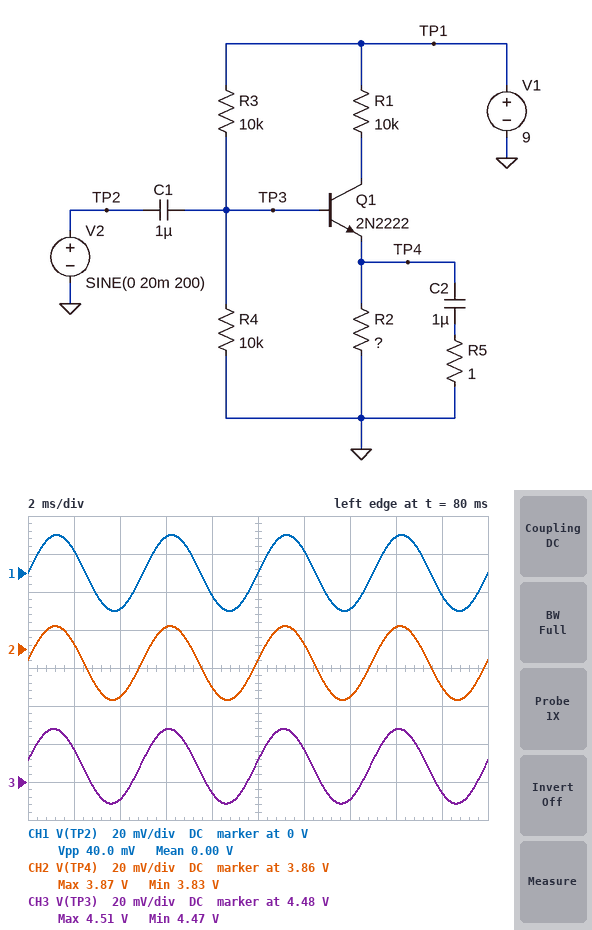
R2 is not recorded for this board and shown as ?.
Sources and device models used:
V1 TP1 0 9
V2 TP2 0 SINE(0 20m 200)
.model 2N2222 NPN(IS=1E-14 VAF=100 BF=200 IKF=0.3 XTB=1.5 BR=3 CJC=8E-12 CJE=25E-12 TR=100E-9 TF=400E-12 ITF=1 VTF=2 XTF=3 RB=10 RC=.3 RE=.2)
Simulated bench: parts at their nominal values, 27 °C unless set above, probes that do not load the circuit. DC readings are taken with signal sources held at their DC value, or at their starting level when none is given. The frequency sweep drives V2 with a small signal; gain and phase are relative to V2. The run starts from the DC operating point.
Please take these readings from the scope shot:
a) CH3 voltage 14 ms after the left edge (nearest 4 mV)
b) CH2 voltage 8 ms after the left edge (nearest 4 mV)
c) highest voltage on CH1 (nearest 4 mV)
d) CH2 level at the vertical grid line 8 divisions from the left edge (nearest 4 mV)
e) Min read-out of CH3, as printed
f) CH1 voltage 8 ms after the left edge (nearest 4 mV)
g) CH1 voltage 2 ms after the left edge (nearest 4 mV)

4.472 V
3.840 V
20 mV
3.872 V
4.47 V
-12 mV
12 mV
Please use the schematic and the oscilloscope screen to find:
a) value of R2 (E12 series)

8.2 kΩ
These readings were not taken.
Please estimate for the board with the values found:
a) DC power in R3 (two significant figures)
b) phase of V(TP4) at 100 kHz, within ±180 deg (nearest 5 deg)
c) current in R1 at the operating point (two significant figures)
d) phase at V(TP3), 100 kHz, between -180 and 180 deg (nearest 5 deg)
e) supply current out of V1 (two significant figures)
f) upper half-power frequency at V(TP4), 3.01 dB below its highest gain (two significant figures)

2.0 mW
-55 deg
470 µA
0 deg
920 µA
2.8 kHz
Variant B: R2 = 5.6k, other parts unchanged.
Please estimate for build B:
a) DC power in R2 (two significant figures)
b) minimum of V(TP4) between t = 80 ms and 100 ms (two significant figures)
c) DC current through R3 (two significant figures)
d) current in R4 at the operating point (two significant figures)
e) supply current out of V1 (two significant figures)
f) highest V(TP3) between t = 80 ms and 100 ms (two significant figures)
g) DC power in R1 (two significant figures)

2.2 mW
3.5 V
490 µA
410 µA
1.0 mA
4.1 V
3.0 mW
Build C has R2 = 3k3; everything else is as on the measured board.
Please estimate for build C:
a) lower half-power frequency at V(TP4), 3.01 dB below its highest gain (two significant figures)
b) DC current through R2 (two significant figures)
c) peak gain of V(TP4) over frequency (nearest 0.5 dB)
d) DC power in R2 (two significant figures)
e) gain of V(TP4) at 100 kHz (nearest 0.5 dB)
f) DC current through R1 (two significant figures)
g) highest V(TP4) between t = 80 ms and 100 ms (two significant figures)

47 Hz
840 µA
-6.0 dB
2.3 mW
-32.5 dB
620 µA
2.8 V
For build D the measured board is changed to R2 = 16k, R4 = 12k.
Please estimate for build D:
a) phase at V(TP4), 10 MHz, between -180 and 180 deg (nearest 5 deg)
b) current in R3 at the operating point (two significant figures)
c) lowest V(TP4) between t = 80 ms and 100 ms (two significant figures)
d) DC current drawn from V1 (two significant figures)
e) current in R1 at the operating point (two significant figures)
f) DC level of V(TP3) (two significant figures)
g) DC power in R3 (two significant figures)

10 deg
410 µA
4.3 V
680 µA
270 µA
4.9 V
1.7 mW
